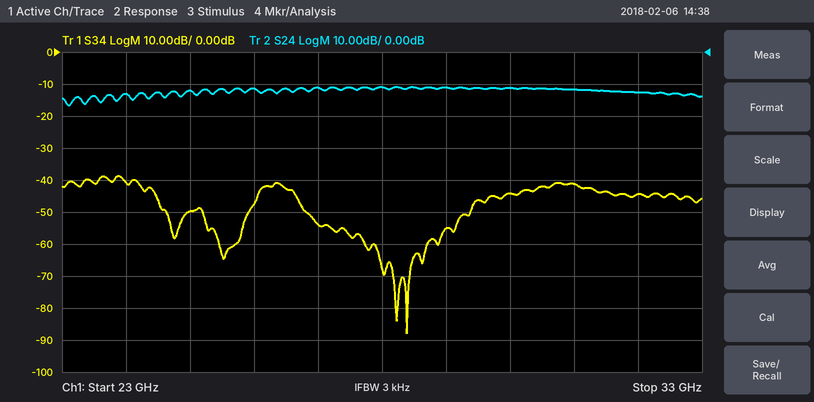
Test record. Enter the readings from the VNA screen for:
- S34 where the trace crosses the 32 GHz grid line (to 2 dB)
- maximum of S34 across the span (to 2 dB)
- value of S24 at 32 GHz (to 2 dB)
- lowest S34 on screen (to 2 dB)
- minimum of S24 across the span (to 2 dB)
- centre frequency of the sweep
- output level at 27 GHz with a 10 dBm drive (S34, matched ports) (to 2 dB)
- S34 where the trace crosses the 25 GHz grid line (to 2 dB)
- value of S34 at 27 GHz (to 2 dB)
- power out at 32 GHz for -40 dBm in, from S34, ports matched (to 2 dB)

-44 dB
-38 dB
-12 dB
-88 dB
-16 dB
28 GHz
-44 dBm
-50 dB
-54 dB
-84 dBm
